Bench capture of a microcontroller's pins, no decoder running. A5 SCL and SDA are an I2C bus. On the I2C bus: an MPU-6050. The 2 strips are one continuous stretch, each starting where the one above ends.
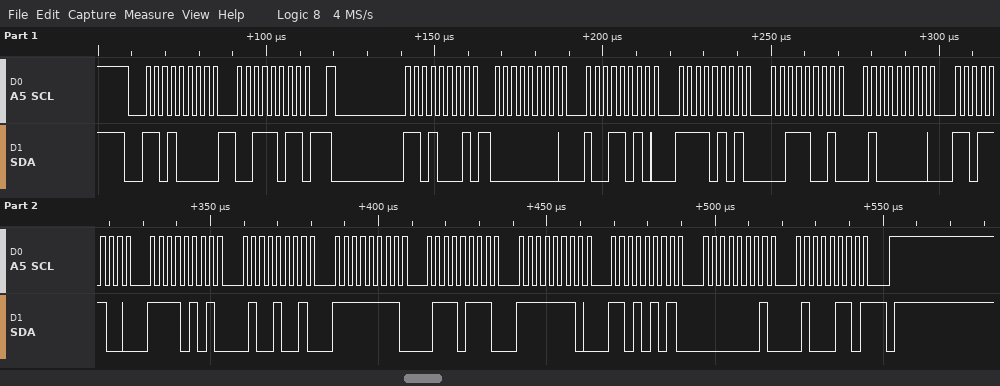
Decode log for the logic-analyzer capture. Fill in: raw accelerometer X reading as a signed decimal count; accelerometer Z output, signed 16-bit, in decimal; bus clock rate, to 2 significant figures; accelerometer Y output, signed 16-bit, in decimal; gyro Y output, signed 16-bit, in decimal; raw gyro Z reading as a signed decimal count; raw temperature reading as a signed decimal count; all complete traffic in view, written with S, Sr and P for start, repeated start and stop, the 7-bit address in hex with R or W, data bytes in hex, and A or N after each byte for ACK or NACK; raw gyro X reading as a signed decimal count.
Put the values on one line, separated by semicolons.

154; 16604; 400 kHz; -2759; -299; 326; -2743; S 68W A 3B A Sr 68R A 00 A 9A A F5 A 39 A 40 A DC A F5 A 49 A FF A 77 A FE A D5 A 01 A 46 N P; -137
